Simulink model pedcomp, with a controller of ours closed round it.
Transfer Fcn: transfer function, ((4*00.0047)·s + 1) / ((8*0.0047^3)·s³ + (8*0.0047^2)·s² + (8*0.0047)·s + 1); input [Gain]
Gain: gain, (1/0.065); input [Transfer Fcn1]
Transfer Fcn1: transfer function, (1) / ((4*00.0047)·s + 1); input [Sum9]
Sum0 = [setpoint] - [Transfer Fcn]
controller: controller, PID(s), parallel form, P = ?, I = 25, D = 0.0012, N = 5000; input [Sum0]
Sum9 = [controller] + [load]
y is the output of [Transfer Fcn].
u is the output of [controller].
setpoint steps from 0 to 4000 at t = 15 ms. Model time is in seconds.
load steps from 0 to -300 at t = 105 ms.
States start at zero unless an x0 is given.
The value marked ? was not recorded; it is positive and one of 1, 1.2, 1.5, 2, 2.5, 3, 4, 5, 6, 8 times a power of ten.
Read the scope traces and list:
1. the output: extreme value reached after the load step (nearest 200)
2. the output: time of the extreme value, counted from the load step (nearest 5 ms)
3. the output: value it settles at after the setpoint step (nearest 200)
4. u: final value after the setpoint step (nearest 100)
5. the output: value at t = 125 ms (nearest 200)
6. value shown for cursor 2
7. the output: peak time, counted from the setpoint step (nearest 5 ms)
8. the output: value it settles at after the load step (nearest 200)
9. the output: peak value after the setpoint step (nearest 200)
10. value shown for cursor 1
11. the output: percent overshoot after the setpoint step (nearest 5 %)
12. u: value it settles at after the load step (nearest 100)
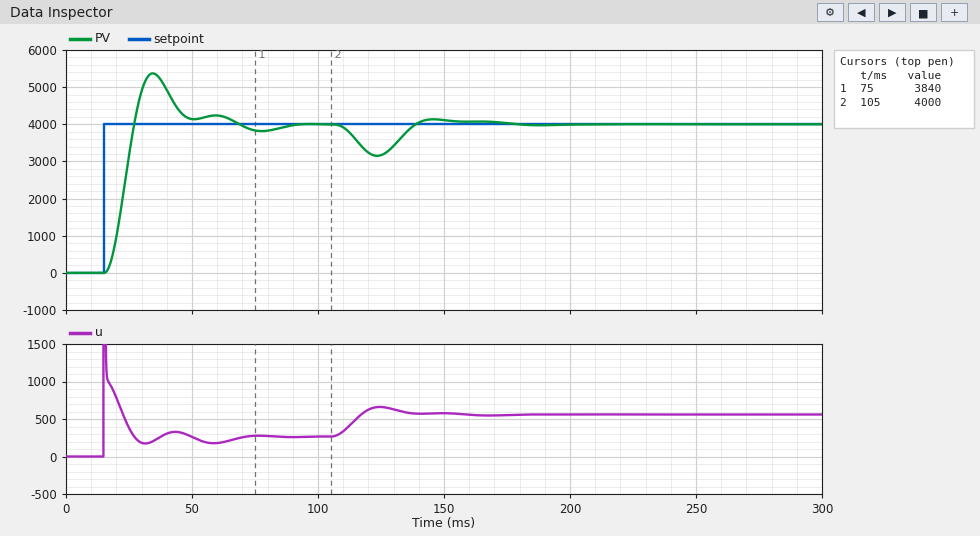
3200
20 ms
4000
300
3200
4000
20 ms
4000
5400
3840
35 %
600
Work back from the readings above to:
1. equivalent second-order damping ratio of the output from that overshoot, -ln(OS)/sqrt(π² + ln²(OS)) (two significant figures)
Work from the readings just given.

0.32
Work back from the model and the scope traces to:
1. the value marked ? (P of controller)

0.25
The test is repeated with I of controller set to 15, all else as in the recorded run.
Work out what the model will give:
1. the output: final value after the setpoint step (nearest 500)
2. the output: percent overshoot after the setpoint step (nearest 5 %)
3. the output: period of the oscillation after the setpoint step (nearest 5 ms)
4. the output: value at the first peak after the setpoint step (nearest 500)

4000
15 %
25 ms
4500
